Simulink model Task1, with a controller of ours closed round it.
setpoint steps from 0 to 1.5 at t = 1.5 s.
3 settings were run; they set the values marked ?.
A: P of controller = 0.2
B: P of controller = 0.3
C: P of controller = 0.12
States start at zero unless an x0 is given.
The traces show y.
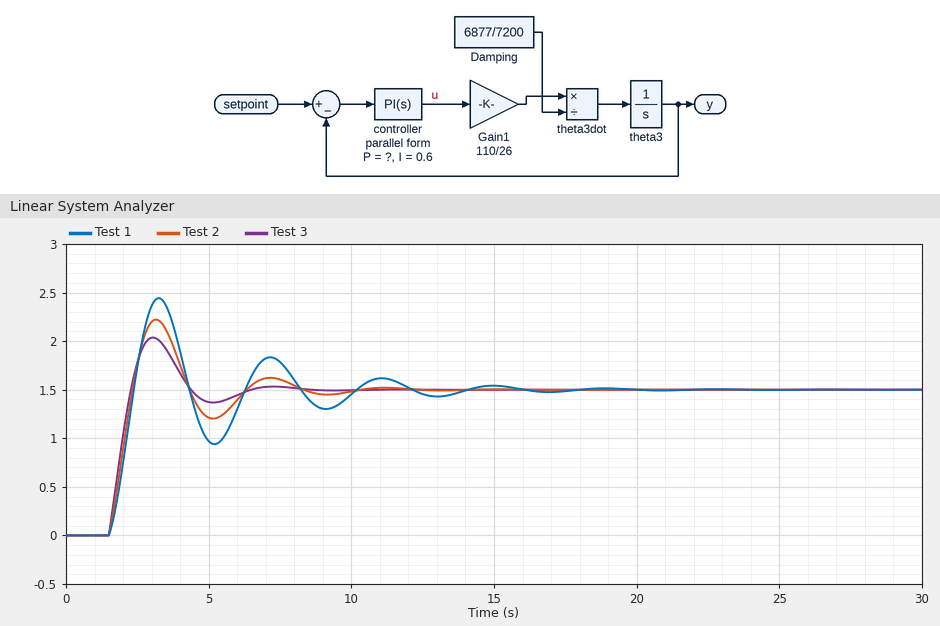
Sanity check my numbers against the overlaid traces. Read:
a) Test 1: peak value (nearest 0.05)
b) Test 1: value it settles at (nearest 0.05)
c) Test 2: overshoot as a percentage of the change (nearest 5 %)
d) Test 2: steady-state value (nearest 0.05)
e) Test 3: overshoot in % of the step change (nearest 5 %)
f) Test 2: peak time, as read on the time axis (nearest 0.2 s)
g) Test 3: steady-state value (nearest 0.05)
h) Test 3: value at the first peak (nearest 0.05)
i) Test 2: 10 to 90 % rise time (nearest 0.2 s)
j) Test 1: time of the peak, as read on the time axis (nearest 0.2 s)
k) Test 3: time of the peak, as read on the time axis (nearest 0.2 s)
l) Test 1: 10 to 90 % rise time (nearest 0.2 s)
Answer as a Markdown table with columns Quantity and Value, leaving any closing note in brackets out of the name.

| Quantity | Value |
|---|---|
| Test 1: peak value | 2.45 |
| Test 1: value it settles at | 1.50 |
| Test 2: overshoot as a percentage of the change | 50 % |
| Test 2: steady-state value | 1.50 |
| Test 3: overshoot in % of the step change | 35 % |
| Test 2: peak time, as read on the time axis | 3.2 s |
| Test 3: steady-state value | 1.50 |
| Test 3: value at the first peak | 2.05 |
| Test 2: 10 to 90 % rise time | 0.6 s |
| Test 1: time of the peak, as read on the time axis | 3.2 s |
| Test 3: time of the peak, as read on the time axis | 3.0 s |
| Test 1: 10 to 90 % rise time | 0.6 s |
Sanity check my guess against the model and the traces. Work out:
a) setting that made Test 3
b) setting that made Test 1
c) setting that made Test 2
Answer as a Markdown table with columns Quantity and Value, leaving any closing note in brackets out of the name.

| Quantity | Value |
|---|---|
| setting that made Test 3 | B |
| setting that made Test 1 | C |
| setting that made Test 2 | A |
